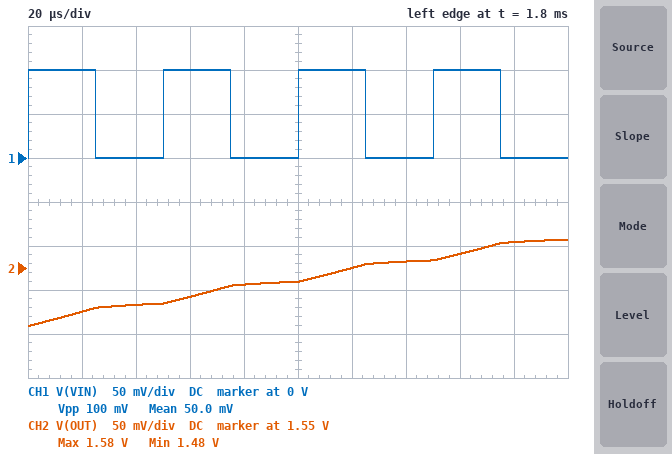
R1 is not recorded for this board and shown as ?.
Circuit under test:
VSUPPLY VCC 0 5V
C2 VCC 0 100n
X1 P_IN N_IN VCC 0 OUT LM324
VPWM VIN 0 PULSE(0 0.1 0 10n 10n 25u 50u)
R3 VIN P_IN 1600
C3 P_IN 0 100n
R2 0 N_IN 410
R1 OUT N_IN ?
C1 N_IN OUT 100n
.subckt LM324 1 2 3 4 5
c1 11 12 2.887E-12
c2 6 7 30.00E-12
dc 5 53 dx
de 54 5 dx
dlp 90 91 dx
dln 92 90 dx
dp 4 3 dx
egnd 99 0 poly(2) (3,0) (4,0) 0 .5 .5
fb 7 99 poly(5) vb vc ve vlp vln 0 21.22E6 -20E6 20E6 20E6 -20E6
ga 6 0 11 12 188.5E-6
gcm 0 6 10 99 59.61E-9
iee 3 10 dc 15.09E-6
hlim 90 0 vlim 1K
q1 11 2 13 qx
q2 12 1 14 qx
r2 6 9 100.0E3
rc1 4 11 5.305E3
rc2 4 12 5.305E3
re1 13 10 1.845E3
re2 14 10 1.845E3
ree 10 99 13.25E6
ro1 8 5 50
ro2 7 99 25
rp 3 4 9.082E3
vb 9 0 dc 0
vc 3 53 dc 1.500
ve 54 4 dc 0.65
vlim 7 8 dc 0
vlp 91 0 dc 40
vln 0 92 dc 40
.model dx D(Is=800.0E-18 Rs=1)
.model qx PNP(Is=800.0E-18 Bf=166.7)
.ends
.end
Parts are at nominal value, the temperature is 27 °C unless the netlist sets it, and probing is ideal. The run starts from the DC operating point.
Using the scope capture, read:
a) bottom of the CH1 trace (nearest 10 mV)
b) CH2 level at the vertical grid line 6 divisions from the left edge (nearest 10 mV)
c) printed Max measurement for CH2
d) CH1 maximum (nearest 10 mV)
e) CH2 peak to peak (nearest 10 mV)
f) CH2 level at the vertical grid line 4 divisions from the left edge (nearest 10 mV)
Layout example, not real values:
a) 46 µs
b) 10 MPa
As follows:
a) 0 V
b) 1.55 V
c) 1.58 V
d) 100 mV
e) 100 mV
f) 1.53 V
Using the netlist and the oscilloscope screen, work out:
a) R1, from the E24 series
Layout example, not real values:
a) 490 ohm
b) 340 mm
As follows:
a) 20 kΩ
